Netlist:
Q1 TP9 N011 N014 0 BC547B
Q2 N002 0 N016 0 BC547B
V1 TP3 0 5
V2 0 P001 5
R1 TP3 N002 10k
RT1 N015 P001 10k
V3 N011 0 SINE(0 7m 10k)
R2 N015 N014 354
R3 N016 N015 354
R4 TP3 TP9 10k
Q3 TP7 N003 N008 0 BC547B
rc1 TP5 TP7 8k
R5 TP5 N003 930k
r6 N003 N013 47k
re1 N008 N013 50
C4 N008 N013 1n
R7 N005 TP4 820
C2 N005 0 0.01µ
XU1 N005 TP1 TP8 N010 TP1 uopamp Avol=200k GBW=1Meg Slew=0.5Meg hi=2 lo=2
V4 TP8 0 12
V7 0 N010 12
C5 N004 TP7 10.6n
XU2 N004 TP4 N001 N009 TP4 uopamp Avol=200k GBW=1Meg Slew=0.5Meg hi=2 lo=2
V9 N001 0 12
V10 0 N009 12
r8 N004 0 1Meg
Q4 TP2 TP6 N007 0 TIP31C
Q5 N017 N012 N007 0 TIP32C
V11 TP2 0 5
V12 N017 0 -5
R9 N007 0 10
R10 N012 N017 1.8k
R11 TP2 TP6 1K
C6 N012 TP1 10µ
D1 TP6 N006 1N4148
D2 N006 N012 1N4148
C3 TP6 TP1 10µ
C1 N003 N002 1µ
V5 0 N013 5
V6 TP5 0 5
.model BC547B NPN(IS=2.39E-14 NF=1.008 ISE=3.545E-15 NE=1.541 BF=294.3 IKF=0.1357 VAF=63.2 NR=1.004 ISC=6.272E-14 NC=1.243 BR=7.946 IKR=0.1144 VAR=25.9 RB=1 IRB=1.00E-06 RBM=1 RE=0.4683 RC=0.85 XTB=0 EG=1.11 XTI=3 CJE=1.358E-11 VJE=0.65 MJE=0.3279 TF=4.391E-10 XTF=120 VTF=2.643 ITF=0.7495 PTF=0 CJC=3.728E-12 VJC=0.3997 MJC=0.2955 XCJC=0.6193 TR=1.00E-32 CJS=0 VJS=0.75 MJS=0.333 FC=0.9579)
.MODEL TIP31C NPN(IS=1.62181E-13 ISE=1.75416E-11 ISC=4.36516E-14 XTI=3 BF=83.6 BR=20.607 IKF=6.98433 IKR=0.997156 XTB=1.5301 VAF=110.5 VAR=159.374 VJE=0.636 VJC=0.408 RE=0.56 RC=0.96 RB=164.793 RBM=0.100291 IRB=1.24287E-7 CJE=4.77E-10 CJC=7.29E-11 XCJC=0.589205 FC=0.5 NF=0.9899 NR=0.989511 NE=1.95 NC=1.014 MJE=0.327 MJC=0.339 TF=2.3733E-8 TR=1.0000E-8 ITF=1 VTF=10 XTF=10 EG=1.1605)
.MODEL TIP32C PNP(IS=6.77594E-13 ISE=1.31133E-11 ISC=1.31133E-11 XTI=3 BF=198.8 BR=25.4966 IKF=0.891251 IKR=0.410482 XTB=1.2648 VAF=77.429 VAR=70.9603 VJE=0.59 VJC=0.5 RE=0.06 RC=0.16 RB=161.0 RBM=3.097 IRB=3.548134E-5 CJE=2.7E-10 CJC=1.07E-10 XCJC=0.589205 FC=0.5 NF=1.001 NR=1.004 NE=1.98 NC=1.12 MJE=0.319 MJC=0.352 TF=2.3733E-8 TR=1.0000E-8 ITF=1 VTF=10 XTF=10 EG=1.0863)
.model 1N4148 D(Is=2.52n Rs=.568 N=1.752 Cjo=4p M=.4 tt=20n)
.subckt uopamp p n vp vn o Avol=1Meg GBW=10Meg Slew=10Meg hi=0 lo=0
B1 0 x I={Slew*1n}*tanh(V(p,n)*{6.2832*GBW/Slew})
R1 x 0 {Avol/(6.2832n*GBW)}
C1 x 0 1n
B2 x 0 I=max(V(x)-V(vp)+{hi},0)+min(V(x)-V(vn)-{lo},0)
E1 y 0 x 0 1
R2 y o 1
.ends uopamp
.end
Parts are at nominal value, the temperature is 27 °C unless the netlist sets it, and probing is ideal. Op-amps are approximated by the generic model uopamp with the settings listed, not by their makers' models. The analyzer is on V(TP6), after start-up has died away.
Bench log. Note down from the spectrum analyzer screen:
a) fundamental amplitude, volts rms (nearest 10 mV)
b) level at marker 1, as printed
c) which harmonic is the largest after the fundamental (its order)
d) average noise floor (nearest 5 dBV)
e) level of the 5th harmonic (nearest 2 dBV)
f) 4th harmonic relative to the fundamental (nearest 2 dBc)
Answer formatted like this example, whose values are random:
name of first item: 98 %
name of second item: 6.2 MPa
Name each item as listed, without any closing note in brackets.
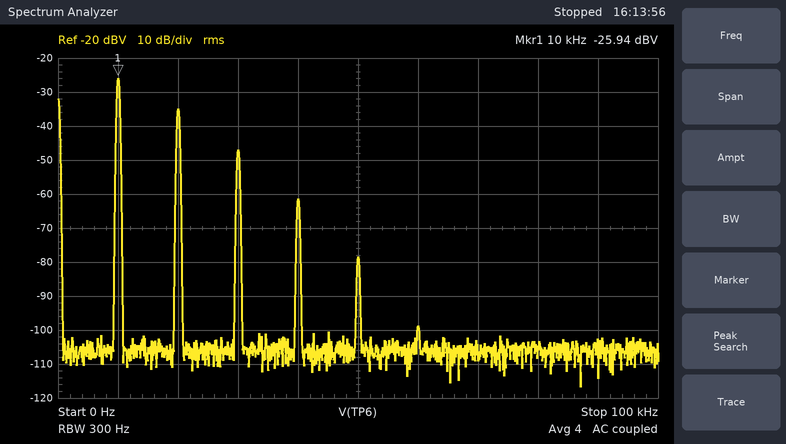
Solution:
fundamental amplitude, volts rms: 50 mV
level at marker 1, as printed: -25.94 dBV
which harmonic is the largest after the fundamental: 2
average noise floor: -105 dBV
level of the 5th harmonic: -78 dBV
4th harmonic relative to the fundamental: -36 dBc
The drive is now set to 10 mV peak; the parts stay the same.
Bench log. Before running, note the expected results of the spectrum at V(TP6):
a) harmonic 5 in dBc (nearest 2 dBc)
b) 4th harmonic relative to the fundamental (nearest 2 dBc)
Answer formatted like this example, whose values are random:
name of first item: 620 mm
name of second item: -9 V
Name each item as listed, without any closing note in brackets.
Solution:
harmonic 5 in dBc: -44 dBc
4th harmonic relative to the fundamental: -30 dBc
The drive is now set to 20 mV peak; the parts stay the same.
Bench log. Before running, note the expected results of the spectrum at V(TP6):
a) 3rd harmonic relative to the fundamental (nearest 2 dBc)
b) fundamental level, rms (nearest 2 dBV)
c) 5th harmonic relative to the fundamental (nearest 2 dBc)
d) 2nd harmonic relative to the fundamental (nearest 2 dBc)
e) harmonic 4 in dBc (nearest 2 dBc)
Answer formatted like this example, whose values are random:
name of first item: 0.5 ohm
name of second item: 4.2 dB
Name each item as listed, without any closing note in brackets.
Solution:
3rd harmonic relative to the fundamental: -14 dBc
fundamental level, rms: -2 dBV
5th harmonic relative to the fundamental: -48 dBc
2nd harmonic relative to the fundamental: -6 dBc
harmonic 4 in dBc: -26 dBc
